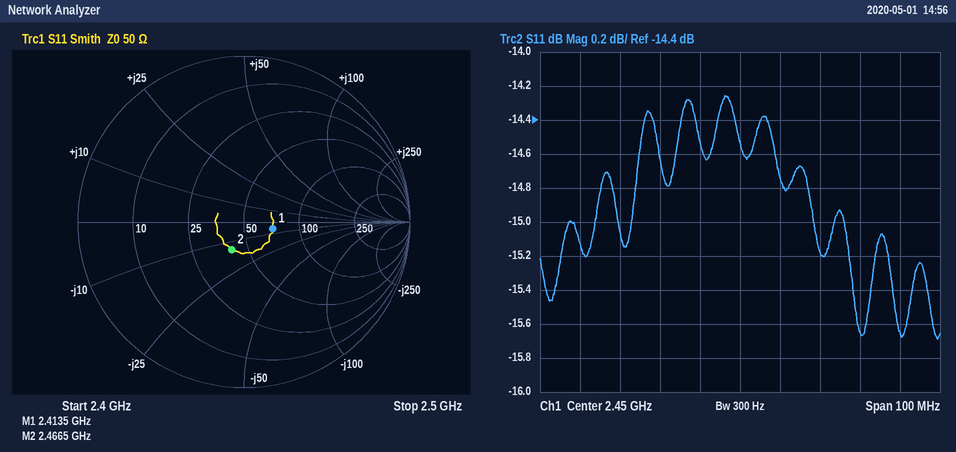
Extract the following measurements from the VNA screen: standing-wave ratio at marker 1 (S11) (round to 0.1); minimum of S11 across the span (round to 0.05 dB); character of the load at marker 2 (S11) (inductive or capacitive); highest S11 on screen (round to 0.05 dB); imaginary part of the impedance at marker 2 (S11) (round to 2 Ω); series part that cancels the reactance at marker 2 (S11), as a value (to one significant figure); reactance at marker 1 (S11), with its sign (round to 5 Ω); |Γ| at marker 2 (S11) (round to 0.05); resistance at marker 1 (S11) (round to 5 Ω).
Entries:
1.4
-15.70 dB
capacitive
-14.25 dB
-14 Ω
900 pH
-5 Ω
0.20
70 Ω
